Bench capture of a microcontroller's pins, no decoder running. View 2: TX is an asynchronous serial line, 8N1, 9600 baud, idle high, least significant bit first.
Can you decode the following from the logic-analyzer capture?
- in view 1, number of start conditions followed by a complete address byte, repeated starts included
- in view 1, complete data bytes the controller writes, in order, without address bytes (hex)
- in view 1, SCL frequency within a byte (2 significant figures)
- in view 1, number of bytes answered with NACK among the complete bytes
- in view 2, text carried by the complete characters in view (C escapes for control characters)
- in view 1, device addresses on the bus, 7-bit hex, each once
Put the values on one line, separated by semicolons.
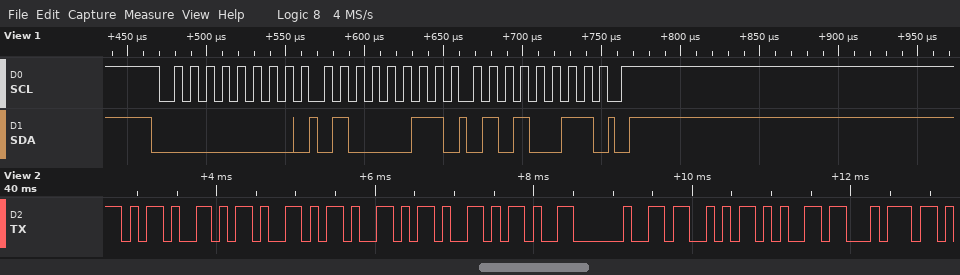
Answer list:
1; 43 53; 100 kHz; 0; "----- Set"; 0x00
